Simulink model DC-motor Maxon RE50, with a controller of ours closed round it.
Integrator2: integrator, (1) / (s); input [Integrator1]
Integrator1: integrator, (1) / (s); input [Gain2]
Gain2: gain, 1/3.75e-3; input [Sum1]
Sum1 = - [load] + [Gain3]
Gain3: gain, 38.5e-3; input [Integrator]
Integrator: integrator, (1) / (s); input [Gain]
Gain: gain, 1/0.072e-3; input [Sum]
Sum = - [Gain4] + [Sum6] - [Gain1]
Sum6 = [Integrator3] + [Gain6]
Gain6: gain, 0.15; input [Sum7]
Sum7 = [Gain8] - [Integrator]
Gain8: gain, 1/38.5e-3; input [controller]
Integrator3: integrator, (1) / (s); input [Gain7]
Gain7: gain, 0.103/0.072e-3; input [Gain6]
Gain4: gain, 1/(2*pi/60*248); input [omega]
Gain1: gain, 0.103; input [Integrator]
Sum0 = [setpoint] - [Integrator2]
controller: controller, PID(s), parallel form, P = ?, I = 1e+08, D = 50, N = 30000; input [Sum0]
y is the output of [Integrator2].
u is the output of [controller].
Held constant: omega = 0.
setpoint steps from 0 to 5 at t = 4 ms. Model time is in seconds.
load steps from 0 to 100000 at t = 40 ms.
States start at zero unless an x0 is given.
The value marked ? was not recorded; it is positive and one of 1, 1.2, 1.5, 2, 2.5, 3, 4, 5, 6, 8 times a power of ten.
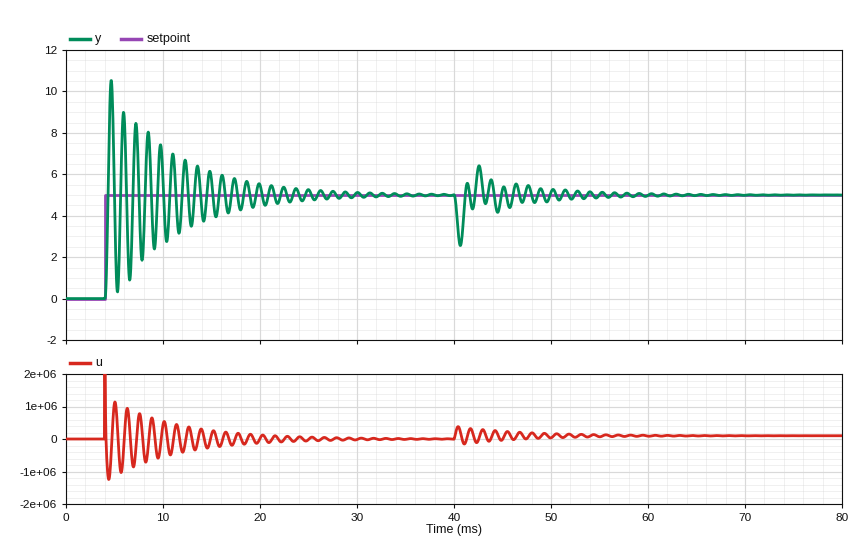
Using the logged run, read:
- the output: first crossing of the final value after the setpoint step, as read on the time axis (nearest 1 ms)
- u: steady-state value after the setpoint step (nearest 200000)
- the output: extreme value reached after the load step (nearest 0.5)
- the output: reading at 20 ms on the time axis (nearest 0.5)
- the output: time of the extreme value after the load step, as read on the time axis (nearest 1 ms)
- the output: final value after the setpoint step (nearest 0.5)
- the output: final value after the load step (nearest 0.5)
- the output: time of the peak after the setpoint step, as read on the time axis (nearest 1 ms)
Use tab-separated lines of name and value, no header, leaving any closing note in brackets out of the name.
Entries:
the output: first crossing of the final value after the setpoint step, as read on the time axis	4 ms
u: steady-state value after the setpoint step	0
the output: extreme value reached after the load step	2.5
the output: reading at 20 ms on the time axis	5.5
the output: time of the extreme value after the load step, as read on the time axis	41 ms
the output: final value after the setpoint step	5.0
the output: final value after the load step	5.0
the output: time of the peak after the setpoint step, as read on the time axis	5 ms
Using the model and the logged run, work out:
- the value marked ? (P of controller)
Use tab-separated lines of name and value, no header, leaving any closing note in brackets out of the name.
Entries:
the value marked ?	40000
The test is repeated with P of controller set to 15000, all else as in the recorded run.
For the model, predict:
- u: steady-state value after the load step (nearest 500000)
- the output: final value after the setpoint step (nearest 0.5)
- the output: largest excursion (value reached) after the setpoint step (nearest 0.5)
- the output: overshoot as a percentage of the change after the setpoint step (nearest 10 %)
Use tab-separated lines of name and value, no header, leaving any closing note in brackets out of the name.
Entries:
u: steady-state value after the load step	0
the output: final value after the setpoint step	5.0
the output: largest excursion (value reached) after the setpoint step	10.0
the output: overshoot as a percentage of the change after the setpoint step	100 %
